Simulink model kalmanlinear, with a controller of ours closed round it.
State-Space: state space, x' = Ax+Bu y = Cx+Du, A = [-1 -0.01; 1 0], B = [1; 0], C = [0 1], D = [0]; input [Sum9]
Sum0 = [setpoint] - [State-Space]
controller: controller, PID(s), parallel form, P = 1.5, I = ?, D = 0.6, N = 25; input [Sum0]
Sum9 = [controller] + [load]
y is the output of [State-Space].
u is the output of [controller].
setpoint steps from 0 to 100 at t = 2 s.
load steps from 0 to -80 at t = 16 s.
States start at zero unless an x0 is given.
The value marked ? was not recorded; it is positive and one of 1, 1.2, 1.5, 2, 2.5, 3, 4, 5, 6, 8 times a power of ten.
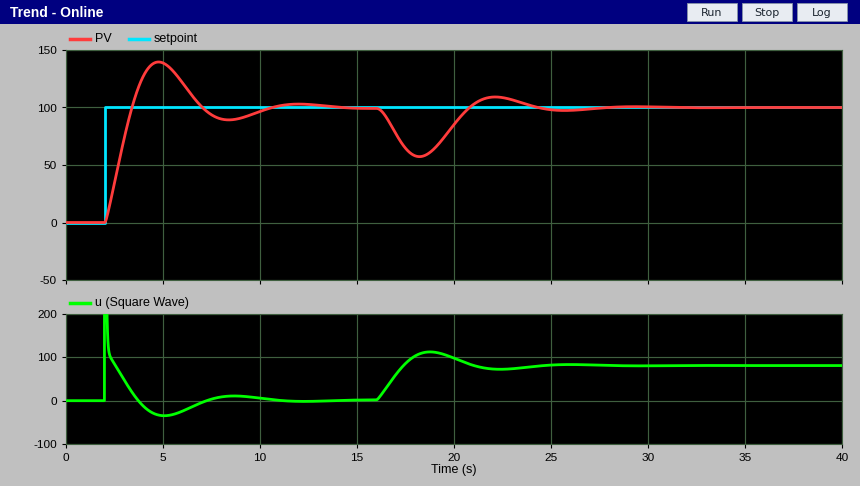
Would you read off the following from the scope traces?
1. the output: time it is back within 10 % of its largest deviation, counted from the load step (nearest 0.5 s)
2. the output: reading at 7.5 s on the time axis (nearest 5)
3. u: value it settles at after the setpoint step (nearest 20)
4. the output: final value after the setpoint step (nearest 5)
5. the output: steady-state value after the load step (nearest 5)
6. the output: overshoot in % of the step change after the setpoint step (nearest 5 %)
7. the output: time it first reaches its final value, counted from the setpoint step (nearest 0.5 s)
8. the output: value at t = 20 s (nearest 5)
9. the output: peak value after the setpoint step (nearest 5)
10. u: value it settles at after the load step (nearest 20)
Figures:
7.5 s
95
0
100
100
40 %
1.5 s
85
140
80
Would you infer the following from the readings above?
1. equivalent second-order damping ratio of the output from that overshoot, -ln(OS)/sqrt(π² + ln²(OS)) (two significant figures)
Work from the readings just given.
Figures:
0.28
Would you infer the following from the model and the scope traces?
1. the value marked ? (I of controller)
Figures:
0.8
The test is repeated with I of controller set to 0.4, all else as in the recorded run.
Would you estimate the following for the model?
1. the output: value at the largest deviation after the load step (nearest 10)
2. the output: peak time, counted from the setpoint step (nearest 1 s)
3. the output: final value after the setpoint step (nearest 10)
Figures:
50
3 s
100
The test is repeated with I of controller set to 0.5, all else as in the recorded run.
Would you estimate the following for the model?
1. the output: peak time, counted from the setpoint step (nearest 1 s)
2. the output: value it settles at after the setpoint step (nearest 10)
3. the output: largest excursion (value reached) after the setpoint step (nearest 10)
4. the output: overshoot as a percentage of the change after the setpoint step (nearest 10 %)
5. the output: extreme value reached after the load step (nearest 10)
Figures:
3 s
100
130
30 %
50
